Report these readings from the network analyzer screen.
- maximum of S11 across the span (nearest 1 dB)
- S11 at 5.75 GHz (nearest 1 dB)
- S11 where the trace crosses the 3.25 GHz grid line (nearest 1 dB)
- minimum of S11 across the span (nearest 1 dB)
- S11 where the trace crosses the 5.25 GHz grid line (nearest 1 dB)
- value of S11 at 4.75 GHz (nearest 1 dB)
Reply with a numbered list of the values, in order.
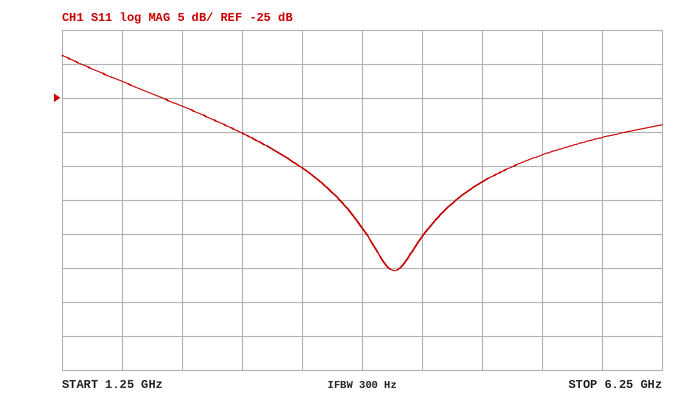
1. -19 dB
2. -31 dB
3. -35 dB
4. -50 dB
5. -33 dB
6. -37 dB
